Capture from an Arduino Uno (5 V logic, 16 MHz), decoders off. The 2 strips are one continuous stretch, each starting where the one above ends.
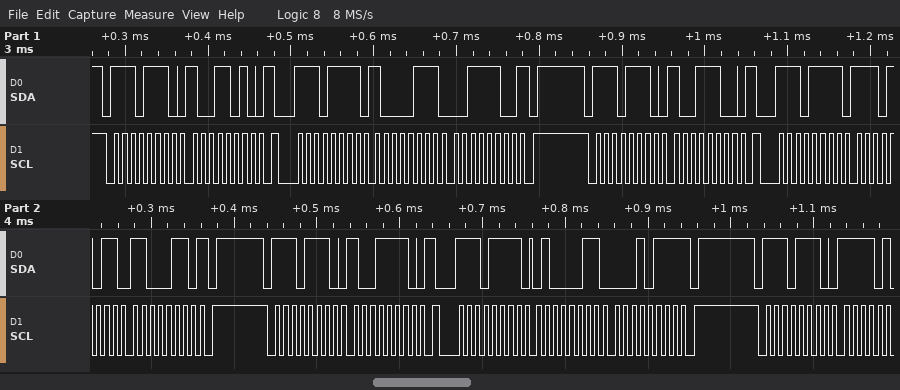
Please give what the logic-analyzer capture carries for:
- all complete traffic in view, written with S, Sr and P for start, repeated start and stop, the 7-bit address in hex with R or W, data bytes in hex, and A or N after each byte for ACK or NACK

S 77W A 9A A Sr 77R A 87 A 3C N P S 77W A 9C A Sr 77R A EB A C6 N P S 77W A 9E A Sr 77R A 43 A 17 N P S 77W A
